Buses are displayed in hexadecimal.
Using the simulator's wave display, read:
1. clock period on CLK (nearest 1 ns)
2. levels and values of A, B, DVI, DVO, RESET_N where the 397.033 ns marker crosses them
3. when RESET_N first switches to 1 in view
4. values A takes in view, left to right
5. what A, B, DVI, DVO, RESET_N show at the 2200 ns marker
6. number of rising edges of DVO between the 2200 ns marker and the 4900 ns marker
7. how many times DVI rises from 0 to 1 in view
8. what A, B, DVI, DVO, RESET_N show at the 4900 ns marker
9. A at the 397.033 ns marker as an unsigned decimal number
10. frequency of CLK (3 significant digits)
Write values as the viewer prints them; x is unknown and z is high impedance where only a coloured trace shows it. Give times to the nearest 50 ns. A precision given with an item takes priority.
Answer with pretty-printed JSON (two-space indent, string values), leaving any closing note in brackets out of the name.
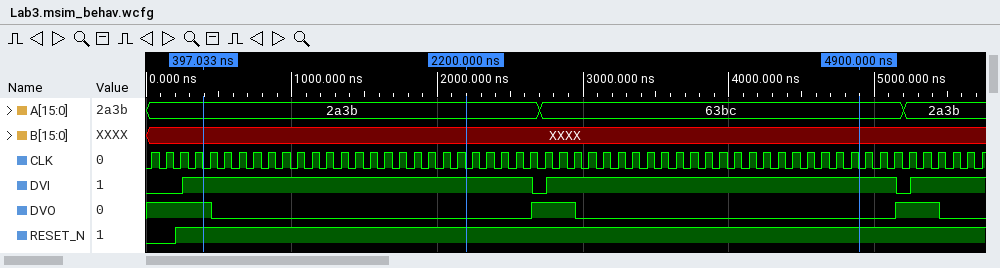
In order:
{
  "clock period on CLK": "100 ns",
  "levels and values of A, B, DVI, DVO, RESET_N where the 397.033 ns marker crosses them": "A=2a3b, B=XXXX, DVI=1, DVO=1, RESET_N=1",
  "when RESET_N first switches to 1 in view": "200 ns",
  "values A takes in view, left to right": "2a3b, 63bc, 2a3b",
  "what A, B, DVI, DVO, RESET_N show at the 2200 ns marker": "A=2a3b, B=XXXX, DVI=1, DVO=0, RESET_N=1",
  "number of rising edges of DVO between the 2200 ns marker and the 4900 ns marker": "1",
  "how many times DVI rises from 0 to 1 in view": "3",
  "what A, B, DVI, DVO, RESET_N show at the 4900 ns marker": "A=63bc, B=XXXX, DVI=1, DVO=0, RESET_N=1",
  "A at the 397.033 ns marker as an unsigned decimal number": "10811",
  "frequency of CLK": "10.0 MHz"
}
